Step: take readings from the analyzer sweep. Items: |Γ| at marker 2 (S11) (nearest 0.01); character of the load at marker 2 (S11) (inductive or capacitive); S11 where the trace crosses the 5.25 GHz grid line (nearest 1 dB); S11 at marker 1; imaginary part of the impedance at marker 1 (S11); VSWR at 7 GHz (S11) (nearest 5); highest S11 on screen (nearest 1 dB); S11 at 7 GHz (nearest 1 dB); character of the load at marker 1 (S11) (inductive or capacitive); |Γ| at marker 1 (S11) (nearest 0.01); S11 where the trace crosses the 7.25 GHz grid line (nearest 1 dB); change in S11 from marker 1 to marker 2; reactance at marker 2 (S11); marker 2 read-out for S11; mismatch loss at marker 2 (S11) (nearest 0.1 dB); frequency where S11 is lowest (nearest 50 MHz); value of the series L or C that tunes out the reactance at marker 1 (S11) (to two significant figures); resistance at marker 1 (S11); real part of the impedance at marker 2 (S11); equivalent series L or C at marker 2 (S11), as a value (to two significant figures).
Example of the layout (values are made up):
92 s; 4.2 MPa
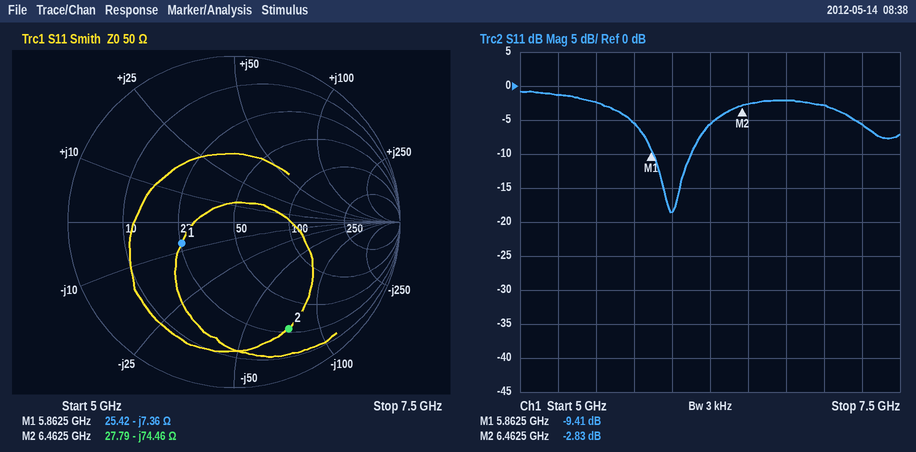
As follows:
0.72; capacitive; -1 dB; -9.41 dB; -7.36 Ω; 5; -1 dB; -3 dB; capacitive; 0.34; -6 dB; 6.58 dB; -74.46 Ω; -2.83 dB; 3.2 dB; 6.00 GHz; 200 pH; 25.42 Ω; 27.79 Ω; 330 fF
